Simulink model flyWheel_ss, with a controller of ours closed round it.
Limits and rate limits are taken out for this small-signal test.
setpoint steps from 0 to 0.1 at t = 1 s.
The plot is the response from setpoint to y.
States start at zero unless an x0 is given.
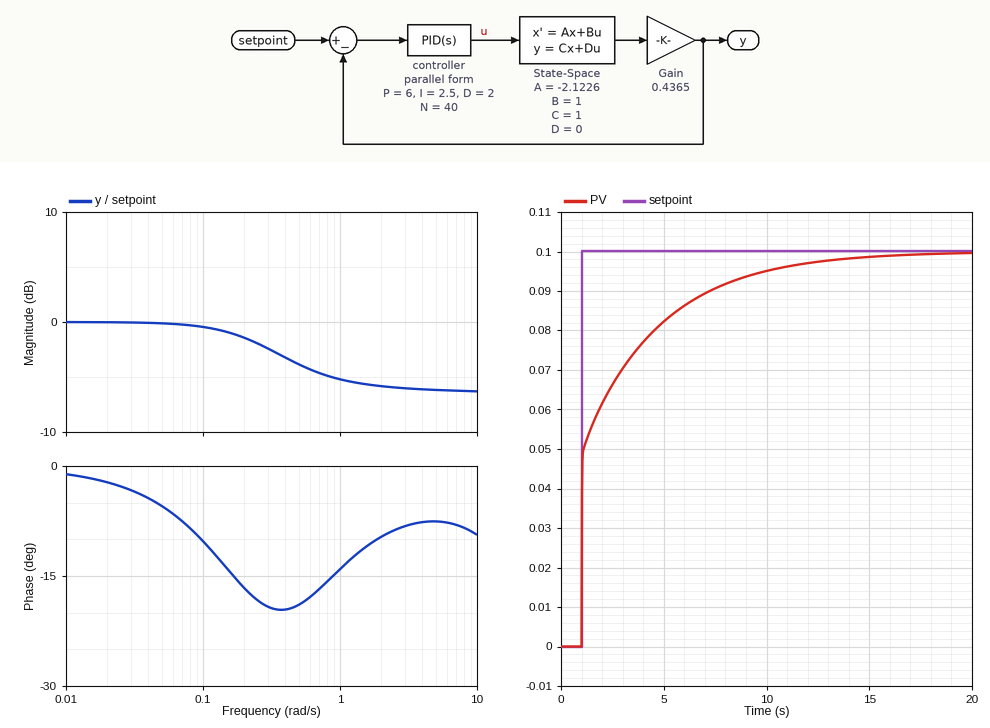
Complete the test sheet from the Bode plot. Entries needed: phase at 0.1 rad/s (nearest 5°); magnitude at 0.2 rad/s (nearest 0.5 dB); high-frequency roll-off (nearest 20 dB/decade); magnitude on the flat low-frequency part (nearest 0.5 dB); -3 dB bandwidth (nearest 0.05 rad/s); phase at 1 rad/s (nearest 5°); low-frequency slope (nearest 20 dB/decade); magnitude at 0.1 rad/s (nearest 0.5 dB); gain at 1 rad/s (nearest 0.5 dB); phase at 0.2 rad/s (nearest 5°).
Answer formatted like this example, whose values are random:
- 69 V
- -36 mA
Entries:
- -10°
- -1.5 dB
- 0 dB/decade
- 0.0 dB
- 0.35 rad/s
- -15°
- 0 dB/decade
- -0.5 dB
- -5.0 dB
- -15°
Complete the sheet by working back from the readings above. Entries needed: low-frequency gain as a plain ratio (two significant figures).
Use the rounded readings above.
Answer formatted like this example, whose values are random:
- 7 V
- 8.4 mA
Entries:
- 1.0
